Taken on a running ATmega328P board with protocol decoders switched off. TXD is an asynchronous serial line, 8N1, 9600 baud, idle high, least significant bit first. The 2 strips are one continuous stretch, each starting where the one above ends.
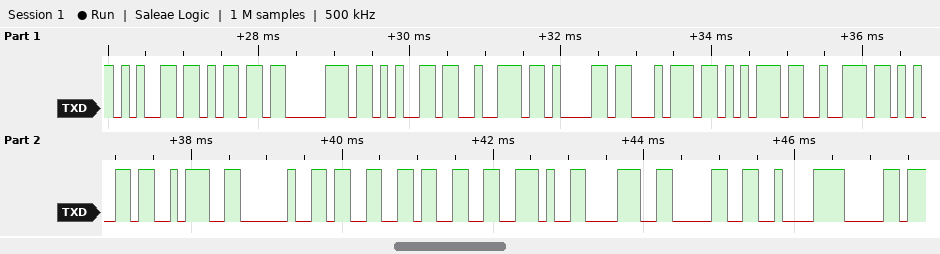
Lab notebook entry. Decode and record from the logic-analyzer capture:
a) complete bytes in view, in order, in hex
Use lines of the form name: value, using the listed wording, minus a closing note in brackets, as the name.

complete bytes in view, in order, in hex: 65 6D 70 65 72 61 74 75 72 65 3A 20 33 33 2E 38 30 C2 B0
